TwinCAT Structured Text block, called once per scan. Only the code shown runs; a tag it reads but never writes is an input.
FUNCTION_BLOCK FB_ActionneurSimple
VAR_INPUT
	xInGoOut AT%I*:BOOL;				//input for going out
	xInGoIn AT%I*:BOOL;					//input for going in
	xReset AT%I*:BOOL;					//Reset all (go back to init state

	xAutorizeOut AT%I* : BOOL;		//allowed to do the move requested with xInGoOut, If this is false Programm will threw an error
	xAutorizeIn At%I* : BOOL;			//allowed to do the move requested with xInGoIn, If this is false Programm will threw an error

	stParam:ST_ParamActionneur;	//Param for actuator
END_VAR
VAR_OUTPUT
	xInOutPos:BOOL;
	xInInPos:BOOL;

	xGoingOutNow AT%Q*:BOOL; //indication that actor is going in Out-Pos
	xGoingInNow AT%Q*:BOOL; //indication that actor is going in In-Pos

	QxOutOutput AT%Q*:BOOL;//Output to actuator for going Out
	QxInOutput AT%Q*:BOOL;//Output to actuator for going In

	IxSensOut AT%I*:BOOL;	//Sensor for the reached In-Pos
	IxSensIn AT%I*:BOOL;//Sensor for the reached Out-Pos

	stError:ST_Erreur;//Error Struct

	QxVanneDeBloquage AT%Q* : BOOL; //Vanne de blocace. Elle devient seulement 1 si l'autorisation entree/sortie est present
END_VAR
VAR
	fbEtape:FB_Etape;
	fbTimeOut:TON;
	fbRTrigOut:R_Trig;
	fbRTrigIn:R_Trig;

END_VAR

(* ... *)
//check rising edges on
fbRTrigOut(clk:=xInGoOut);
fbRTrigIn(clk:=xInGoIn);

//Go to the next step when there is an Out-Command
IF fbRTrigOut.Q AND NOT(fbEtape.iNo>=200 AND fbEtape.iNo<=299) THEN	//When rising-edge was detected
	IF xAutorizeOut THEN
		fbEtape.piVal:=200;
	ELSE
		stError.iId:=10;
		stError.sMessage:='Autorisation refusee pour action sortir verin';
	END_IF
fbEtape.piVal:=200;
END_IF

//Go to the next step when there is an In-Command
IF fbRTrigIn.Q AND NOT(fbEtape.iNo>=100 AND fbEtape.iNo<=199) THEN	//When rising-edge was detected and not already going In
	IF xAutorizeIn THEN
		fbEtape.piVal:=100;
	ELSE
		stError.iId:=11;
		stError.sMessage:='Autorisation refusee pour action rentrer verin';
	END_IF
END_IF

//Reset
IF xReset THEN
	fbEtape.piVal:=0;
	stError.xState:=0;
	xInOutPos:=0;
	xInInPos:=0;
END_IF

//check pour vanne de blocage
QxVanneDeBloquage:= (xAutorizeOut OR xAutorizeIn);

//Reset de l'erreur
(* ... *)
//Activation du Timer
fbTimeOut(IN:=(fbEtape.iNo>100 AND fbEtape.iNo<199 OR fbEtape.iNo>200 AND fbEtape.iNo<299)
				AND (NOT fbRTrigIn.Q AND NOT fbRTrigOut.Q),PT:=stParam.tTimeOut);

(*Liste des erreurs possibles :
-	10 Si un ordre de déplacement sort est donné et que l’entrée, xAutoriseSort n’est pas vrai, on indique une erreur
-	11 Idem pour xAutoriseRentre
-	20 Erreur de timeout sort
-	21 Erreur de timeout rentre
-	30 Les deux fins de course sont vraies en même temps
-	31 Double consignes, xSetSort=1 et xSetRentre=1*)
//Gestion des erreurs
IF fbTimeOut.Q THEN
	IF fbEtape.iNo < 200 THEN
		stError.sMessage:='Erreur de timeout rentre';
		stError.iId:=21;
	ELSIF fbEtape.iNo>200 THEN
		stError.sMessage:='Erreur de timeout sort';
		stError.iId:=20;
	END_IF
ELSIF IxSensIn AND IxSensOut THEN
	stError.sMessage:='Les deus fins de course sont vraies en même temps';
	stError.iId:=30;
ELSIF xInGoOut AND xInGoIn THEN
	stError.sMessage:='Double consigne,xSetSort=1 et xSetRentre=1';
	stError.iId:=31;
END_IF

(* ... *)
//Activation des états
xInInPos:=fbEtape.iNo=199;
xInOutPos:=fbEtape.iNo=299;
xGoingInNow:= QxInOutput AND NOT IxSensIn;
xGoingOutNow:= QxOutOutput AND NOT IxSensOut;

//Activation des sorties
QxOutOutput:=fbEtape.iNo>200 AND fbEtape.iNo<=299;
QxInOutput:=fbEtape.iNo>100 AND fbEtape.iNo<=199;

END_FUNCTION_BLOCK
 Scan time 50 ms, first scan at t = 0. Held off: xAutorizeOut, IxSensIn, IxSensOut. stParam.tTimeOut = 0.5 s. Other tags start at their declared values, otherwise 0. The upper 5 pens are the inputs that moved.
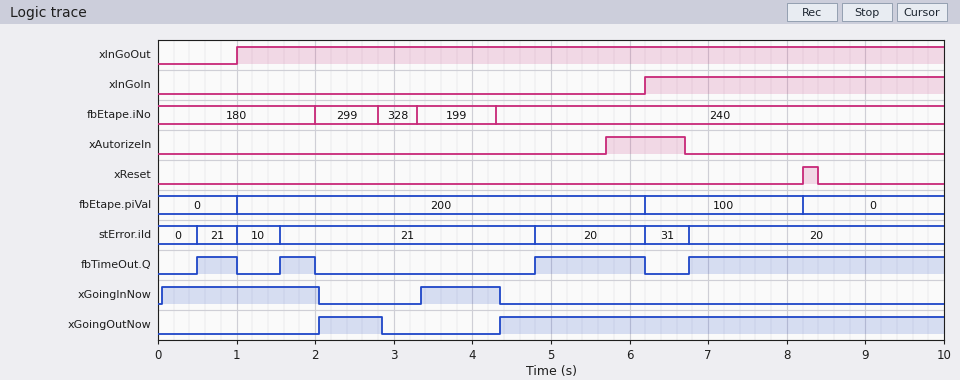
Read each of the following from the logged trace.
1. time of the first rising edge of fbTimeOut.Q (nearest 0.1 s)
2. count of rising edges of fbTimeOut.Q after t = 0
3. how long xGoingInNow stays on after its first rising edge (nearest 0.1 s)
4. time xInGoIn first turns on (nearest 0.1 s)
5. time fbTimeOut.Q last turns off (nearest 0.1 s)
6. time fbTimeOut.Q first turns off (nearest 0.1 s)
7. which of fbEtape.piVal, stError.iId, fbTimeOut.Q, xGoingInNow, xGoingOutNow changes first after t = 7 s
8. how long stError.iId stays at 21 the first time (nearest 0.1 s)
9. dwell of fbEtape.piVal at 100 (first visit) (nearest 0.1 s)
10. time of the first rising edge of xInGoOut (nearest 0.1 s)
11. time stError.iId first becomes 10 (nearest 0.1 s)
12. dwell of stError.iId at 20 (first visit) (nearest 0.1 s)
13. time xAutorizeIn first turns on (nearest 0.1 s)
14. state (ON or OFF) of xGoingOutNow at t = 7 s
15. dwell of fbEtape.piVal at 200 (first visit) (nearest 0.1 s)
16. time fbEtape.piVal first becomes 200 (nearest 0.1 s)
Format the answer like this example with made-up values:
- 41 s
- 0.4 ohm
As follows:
- 0.5 s
- 4
- 2.0 s
- 6.2 s
- 6.2 s
- 1.0 s
- fbEtape.piVal
- 0.5 s
- 2.0 s
- 1.0 s
- 1.0 s
- 1.4 s
- 5.7 s
- ON
- 5.2 s
- 1.0 s
